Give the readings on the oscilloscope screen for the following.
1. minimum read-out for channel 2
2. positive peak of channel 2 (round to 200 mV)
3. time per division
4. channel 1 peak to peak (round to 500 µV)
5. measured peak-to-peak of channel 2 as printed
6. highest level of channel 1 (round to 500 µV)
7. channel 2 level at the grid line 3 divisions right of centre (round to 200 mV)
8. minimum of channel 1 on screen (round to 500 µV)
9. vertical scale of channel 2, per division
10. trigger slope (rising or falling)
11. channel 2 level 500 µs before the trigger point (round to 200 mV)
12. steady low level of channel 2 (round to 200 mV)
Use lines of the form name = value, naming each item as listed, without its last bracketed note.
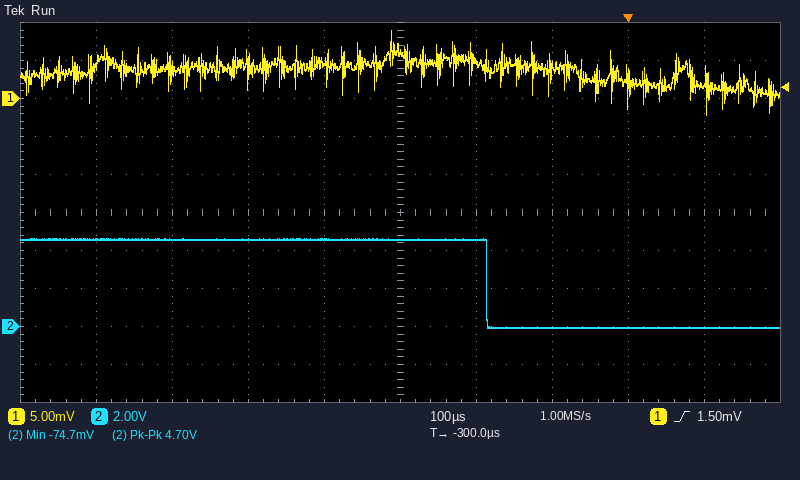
minimum read-out for channel 2 = -74.7 mV
positive peak of channel 2 = 4.6 V
time per division = 100 µs
channel 1 peak to peak = 11.0 mV
measured peak-to-peak of channel 2 as printed = 4.70 V
highest level of channel 1 = 9.0 mV
channel 2 level at the grid line 3 divisions right of centre = 0.0 V
minimum of channel 1 on screen = -2.0 mV
vertical scale of channel 2, per division = 2 V
trigger slope = rising
channel 2 level 500 µs before the trigger point = 4.6 V
steady low level of channel 2 = 0.0 V
